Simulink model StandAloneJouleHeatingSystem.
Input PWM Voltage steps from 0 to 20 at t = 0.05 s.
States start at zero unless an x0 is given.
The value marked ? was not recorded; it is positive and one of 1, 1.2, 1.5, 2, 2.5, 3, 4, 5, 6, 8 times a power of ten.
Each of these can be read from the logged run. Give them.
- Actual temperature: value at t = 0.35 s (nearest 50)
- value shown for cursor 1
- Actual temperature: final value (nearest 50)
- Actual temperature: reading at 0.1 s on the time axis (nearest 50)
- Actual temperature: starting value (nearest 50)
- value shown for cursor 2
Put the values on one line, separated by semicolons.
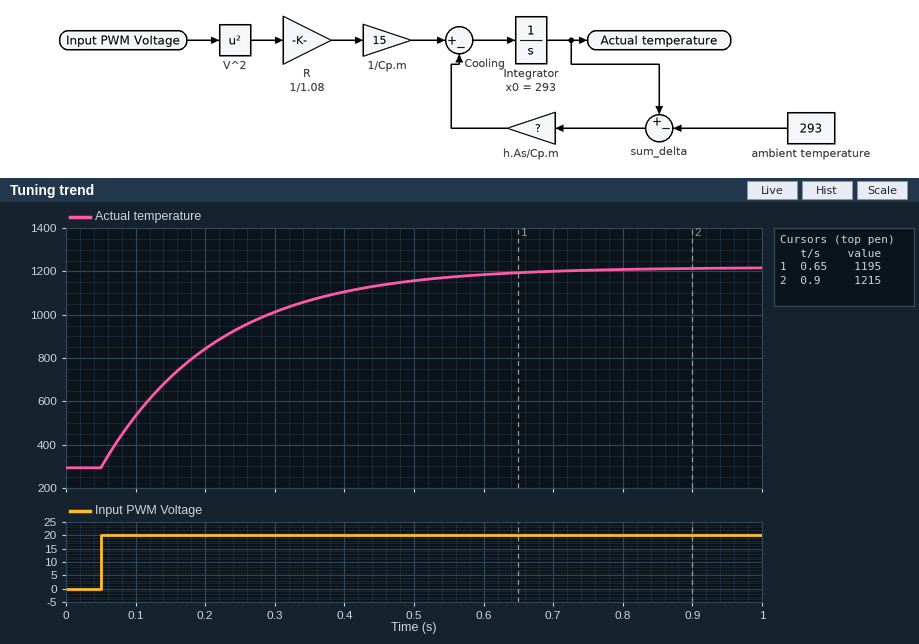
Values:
1050; 1195; 1200; 550; 300; 1215
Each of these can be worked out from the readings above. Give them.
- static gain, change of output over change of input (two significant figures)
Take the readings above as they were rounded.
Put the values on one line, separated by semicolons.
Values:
45
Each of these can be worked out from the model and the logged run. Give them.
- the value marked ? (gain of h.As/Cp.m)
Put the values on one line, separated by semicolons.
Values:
6
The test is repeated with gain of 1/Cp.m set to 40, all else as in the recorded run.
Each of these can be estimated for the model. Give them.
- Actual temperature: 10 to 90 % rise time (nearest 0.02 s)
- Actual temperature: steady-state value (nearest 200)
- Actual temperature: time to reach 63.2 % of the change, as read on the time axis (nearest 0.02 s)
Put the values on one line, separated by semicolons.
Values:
0.36 s; 2800; 0.22 s
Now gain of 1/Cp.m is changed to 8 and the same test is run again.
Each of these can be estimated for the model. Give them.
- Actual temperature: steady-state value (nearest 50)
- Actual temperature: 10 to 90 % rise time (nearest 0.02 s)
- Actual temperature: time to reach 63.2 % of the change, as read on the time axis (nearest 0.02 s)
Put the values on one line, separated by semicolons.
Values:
800; 0.36 s; 0.22 s
